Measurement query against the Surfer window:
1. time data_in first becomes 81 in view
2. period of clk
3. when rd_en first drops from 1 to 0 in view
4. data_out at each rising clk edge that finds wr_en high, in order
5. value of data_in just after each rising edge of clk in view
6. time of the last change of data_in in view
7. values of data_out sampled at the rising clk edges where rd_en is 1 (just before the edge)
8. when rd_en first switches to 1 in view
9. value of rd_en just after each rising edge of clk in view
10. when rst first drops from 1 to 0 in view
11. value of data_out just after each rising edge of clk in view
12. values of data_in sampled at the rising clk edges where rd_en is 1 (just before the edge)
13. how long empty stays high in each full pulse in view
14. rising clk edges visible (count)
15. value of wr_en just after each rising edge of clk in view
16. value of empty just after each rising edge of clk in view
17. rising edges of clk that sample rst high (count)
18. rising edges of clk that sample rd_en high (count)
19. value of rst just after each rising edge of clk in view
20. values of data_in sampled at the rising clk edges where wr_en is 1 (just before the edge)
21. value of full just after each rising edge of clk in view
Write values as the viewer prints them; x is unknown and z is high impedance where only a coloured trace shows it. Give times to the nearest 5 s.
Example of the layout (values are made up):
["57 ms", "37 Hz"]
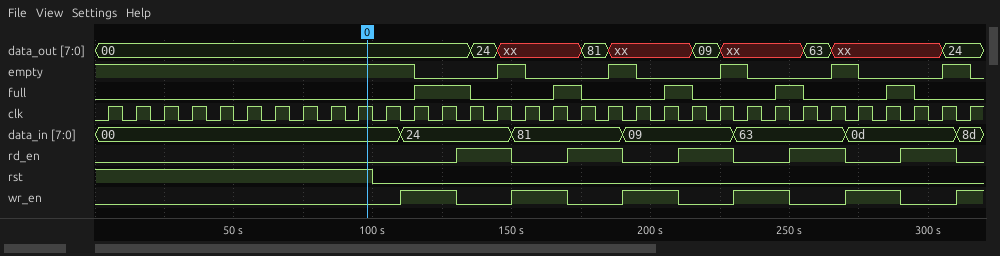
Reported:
["150 s", "10 s", "150 s", "00, 00, xx, xx, xx, xx, xx, xx, xx, xx, 24", "00, 00, 00, 00, 00, 00, 00, 00, 00, 00, 00, 24, 24, 24, 24, 81, 81, 81, 81, 09, 09, 09, 09, 63, 63, 63, 63, 0d, 0d, 0d, 0d, 8d", "310 s", "00, 24, xx, 81, xx, 09, xx, 63, xx, xx", "130 s", "0 0 0 0 0 0 0 0 0 0 0 0 0 1 1 0 0 1 1 0 0 1 1 0 0 1 1 0 0 1 1 0", "100 s", "00, 00, 00, 00, 00, 00, 00, 00, 00, 00, 00, 00, 00, 24, xx, xx, xx, 81, xx, xx, xx, 09, xx, xx, xx, 63, xx, xx, xx, xx, 24, 24", "24, 24, 81, 81, 09, 09, 63, 63, 0d, 0d", "10 s, 10 s, 10 s, 10 s, 10 s", "32", "0 0 0 0 0 0 0 0 0 0 0 1 1 0 0 1 1 0 0 1 1 0 0 1 1 0 0 1 1 0 0 1", "1 1 1 1 1 1 1 1 1 1 1 0 0 0 1 0 0 0 1 0 0 0 1 0 0 0 1 0 0 0 1 0", "10", "10", "1 1 1 1 1 1 1 1 1 1 0 0 0 0 0 0 0 0 0 0 0 0 0 0 0 0 0 0 0 0 0 0", "24, 24, 81, 81, 09, 09, 63, 63, 0d, 0d, 8d", "0 0 0 0 0 0 0 0 0 0 0 1 1 0 0 0 1 0 0 0 1 0 0 0 1 0 0 0 1 0 0 0"]
